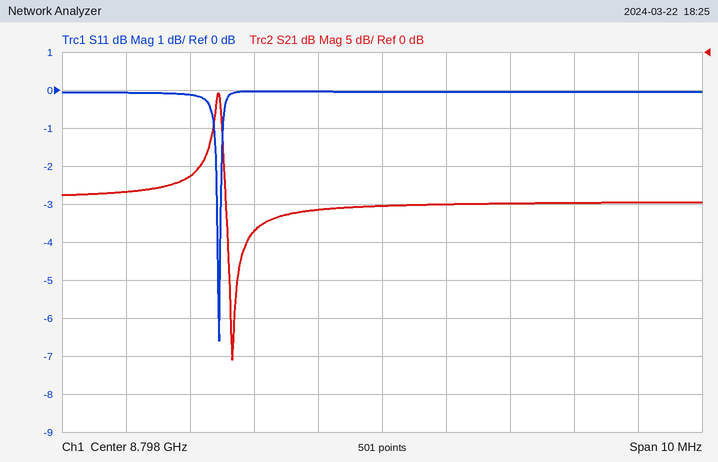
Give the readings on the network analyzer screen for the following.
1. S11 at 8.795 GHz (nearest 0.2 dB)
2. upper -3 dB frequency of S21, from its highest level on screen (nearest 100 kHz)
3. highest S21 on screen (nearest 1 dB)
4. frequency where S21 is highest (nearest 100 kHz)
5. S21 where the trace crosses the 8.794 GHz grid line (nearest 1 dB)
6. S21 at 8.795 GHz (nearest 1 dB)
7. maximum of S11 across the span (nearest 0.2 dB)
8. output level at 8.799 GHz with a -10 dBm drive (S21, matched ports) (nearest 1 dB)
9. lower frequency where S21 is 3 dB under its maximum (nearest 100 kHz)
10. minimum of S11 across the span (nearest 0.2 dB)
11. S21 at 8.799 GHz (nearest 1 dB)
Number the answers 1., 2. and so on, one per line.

1. -0.2 dB
2. 8.7955 GHz
3. -5 dB
4. 8.7954 GHz
5. -18 dB
6. -16 dB
7. 0.0 dB
8. -30 dBm
9. 8.7954 GHz
10. -6.6 dB
11. -20 dB
